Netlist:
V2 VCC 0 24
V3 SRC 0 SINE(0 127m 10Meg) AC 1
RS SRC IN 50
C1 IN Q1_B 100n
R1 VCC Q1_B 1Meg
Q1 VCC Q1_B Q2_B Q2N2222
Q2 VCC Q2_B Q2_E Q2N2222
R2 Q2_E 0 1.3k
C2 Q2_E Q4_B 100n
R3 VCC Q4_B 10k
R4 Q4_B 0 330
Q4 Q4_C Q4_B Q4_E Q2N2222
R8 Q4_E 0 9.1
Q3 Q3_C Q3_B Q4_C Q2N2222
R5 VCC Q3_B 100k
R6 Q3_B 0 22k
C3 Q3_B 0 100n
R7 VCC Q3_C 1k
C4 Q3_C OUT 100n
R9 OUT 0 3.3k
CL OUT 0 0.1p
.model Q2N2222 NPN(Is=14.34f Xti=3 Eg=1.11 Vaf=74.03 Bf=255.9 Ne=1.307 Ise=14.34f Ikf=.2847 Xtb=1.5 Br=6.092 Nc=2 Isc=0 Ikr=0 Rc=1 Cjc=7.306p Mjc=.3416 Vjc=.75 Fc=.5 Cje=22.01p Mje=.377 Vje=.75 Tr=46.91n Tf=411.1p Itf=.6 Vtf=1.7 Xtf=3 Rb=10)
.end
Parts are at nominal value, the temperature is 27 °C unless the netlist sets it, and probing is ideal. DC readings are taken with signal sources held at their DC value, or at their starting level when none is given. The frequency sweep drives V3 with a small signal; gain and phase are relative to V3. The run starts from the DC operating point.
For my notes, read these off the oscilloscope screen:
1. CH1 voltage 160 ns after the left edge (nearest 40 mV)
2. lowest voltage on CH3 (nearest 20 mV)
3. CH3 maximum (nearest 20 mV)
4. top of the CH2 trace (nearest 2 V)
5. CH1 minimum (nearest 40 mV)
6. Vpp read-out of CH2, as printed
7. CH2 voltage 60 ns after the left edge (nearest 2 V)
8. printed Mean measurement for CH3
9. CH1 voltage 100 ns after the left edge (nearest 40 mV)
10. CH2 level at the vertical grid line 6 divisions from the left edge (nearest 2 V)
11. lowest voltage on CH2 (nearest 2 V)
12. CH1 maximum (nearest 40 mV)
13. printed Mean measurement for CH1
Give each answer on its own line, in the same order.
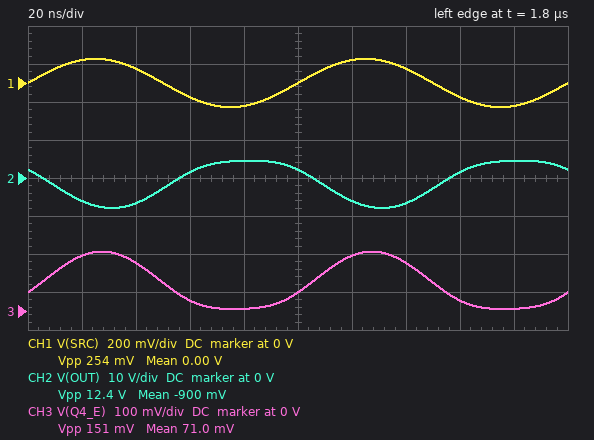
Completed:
-80 mV
0 V
160 mV
4 V
-120 mV
12.4 V
2 V
71.0 mV
0 V
-6 V
-8 V
120 mV
0.00 V
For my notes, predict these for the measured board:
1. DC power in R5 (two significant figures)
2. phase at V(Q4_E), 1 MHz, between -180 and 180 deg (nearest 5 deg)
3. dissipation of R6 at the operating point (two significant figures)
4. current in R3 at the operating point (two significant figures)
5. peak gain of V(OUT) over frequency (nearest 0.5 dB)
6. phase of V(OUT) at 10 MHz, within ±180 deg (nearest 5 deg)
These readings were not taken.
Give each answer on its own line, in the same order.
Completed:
4.1 mW
0 deg
640 µW
2.3 mA
35.0 dB
160 deg
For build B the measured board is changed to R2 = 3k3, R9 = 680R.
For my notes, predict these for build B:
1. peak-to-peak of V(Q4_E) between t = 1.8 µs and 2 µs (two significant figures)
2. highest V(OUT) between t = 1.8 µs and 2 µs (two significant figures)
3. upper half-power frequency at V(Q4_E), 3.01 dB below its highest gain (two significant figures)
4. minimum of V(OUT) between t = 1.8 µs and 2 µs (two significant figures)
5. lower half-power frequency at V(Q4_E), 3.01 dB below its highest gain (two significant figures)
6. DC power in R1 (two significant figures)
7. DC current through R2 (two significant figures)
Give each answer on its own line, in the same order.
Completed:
140 mV
2.3 V
66 MHz
-3.9 V
5.5 kHz
150 nW
6.8 mA
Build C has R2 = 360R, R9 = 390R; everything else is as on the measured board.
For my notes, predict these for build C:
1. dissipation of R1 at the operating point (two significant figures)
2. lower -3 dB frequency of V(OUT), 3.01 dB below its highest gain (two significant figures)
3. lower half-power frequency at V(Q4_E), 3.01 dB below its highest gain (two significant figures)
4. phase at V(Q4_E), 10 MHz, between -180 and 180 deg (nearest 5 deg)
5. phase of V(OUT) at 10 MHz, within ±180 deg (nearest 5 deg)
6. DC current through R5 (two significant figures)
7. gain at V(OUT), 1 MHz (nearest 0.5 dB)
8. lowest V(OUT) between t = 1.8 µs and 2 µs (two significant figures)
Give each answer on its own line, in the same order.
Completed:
5.5 µW
5.9 kHz
6.1 kHz
-5 deg
170 deg
200 µA
26.5 dB
-3.0 V
